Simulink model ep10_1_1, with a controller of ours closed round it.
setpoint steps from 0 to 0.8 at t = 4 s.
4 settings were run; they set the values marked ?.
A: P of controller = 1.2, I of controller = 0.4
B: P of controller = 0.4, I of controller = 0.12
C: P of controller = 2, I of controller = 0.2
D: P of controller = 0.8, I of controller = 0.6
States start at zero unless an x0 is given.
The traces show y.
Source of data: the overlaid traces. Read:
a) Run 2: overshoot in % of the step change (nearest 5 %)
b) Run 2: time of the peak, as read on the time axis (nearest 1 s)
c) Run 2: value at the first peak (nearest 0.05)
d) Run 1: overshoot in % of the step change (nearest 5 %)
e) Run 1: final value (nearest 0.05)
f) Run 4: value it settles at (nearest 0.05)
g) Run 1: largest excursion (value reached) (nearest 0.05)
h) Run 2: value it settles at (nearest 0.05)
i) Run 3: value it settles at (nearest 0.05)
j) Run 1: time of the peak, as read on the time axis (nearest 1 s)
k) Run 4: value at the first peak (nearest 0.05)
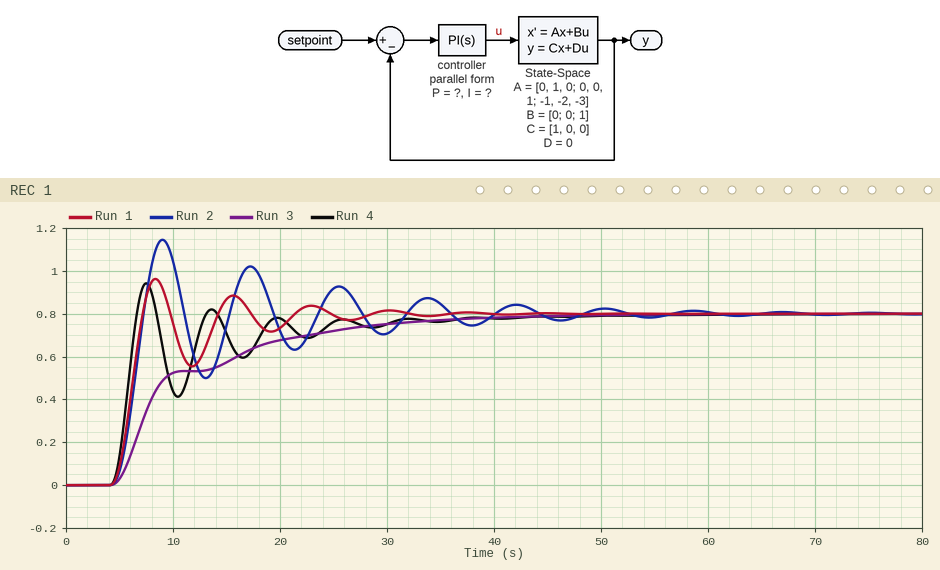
45 %
9 s
1.15
20 %
0.80
0.80
0.95
0.80
0.80
8 s
0.95
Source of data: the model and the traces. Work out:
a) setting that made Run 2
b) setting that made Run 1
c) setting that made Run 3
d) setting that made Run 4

D
A
B
C
